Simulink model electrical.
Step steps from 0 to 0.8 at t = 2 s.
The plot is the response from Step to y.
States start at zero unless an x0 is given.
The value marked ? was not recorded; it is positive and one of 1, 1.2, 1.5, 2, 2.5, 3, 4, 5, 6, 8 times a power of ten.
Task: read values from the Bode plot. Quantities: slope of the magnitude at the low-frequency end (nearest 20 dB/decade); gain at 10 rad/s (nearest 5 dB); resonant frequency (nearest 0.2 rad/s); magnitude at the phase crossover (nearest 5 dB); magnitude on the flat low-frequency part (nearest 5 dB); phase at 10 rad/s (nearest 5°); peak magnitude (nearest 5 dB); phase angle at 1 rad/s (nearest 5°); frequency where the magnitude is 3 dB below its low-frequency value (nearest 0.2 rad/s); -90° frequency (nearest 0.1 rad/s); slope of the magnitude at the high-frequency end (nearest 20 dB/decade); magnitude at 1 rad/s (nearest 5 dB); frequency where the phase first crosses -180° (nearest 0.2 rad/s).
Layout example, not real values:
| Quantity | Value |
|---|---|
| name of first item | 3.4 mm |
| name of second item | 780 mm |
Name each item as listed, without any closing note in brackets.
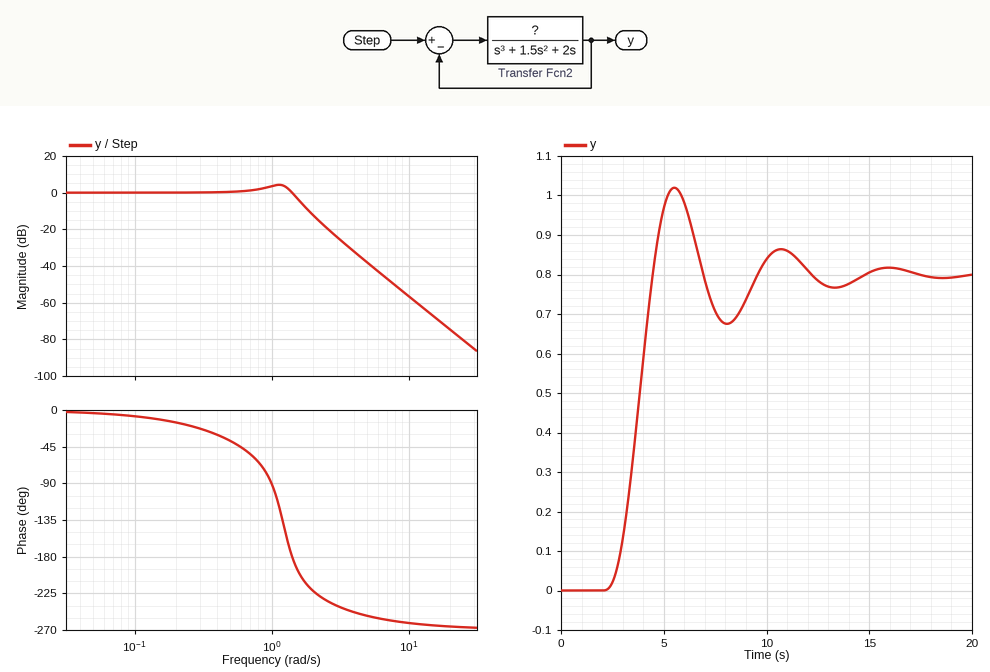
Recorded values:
| Quantity | Value |
|---|---|
| slope of the magnitude at the low-frequency end | 0 dB/decade |
| gain at 10 rad/s | -55 dB |
| resonant frequency | 1.2 rad/s |
| magnitude at the phase crossover | 0 dB |
| magnitude on the flat low-frequency part | 0 dB |
| phase at 10 rad/s | -260° |
| peak magnitude | 5 dB |
| phase angle at 1 rad/s | -90° |
| frequency where the magnitude is 3 dB below its low-frequency value | 1.6 rad/s |
| -90° frequency | 1.0 rad/s |
| slope of the magnitude at the high-frequency end | -60 dB/decade |
| magnitude at 1 rad/s | 5 dB |
| frequency where the phase first crosses -180° | 1.4 rad/s |
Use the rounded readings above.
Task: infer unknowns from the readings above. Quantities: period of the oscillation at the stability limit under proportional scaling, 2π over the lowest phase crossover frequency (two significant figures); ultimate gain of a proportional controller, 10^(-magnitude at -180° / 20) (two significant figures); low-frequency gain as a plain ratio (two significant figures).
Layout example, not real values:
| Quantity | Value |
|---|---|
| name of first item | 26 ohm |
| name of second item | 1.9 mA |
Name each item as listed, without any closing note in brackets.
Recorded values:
| Quantity | Value |
|---|---|
| period of the oscillation at the stability limit under proportional scaling, 2π over the lowest phase crossover frequency | 4.5 s |
| ultimate gain of a proportional controller, 10^(-magnitude at -180° / 20) | 1.0 |
| low-frequency gain as a plain ratio | 1.0 |
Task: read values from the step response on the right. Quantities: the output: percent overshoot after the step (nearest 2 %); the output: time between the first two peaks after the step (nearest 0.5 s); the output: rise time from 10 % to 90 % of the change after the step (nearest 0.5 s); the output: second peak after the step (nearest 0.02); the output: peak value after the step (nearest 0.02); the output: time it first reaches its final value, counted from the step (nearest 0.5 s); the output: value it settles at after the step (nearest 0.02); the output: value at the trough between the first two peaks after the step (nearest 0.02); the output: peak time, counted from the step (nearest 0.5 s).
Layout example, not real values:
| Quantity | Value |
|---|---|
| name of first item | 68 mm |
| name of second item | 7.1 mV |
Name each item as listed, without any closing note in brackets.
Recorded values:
| Quantity | Value |
|---|---|
| the output: percent overshoot after the step | 28 % |
| the output: time between the first two peaks after the step | 5.0 s |
| the output: rise time from 10 % to 90 % of the change after the step | 1.5 s |
| the output: second peak after the step | 0.86 |
| the output: peak value after the step | 1.02 |
| the output: time it first reaches its final value, counted from the step | 2.5 s |
| the output: value it settles at after the step | 0.80 |
| the output: value at the trough between the first two peaks after the step | 0.68 |
| the output: peak time, counted from the step | 3.5 s |
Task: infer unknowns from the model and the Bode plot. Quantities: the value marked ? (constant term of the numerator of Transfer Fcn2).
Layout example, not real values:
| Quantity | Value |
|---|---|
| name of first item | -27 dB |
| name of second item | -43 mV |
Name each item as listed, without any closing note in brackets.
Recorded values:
| Quantity | Value |
|---|---|
| the value marked ? | 1.5 |
